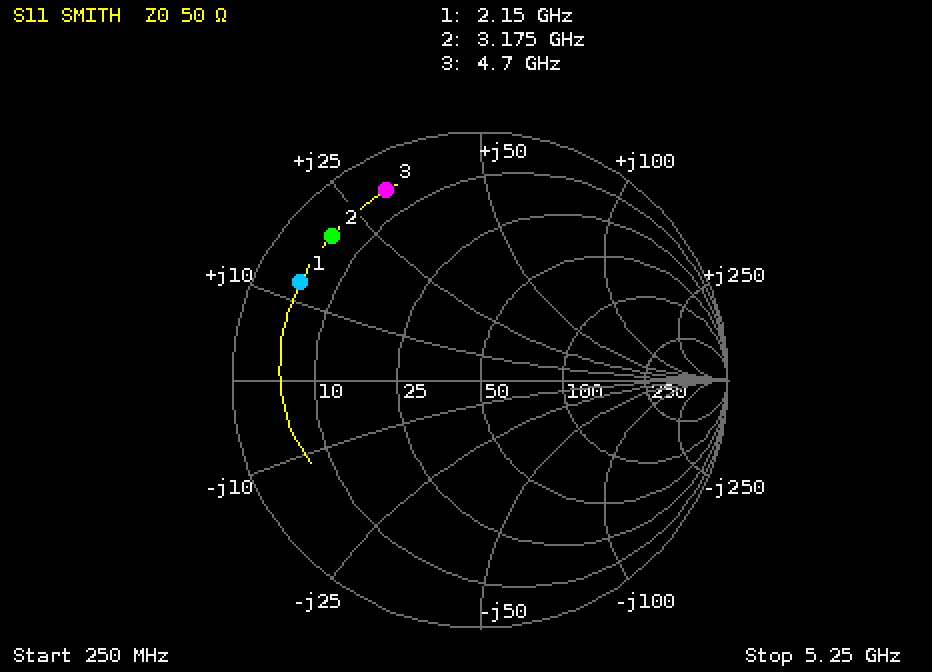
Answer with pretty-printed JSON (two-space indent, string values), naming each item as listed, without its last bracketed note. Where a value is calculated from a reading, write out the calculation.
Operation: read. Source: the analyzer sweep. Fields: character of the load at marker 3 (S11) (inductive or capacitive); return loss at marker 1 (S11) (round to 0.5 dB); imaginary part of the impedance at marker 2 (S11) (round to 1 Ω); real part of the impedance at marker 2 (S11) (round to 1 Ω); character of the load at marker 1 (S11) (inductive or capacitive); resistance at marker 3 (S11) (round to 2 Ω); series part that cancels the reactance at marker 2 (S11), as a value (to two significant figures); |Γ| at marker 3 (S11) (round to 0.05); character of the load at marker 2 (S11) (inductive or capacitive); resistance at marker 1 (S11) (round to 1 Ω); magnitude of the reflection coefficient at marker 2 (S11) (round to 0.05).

{
  "character of the load at marker 3 (S11)": "inductive",
  "return loss at marker 1 (S11)": "1.5 dB",
  "imaginary part of the impedance at marker 2 (S11)": "+20 Ω",
  "real part of the impedance at marker 2 (S11)": "5 Ω",
  "character of the load at marker 1 (S11)": "inductive",
  "resistance at marker 3 (S11)": "6 Ω",
  "series part that cancels the reactance at marker 2 (S11), as a value": "C = 1/(2π × 3.175 GHz × 20 Ω) ≈ 2.5 pF",
  "|Γ| at marker 3 (S11)": "0.85",
  "character of the load at marker 2 (S11)": "inductive",
  "resistance at marker 1 (S11)": "5 Ω",
  "magnitude of the reflection coefficient at marker 2 (S11)": "0.85"
}
